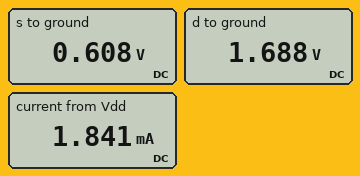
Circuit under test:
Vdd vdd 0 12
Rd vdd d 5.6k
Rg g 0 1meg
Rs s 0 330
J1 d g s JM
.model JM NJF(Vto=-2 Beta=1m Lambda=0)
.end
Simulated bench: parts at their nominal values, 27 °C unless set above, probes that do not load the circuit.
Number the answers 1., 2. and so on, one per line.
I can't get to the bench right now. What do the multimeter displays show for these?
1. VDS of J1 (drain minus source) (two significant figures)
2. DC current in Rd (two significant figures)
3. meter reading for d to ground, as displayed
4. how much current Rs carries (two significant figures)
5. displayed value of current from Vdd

1. 1.1 V
2. 1.8 mA
3. 1.688 V
4. 1.8 mA
5. 1.841 mA
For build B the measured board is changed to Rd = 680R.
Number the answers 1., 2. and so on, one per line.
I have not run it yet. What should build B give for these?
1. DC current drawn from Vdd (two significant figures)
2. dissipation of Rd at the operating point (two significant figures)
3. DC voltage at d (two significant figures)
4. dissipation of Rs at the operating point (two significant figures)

1. 1.9 mA
2. 2.4 mW
3. 11 V
4. 1.2 mW
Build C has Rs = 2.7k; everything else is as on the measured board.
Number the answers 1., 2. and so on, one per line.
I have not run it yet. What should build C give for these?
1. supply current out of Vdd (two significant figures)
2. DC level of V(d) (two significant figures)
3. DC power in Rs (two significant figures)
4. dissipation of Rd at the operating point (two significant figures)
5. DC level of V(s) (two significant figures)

1. 480 µA
2. 9.3 V
3. 630 µW
4. 1.3 mW
5. 1.3 V
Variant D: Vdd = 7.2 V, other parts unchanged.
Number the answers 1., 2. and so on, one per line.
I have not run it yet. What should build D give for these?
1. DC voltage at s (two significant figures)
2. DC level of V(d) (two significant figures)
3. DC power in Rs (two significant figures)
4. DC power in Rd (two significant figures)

1. 380 mV
2. 780 mV
3. 430 µW
4. 7.4 mW
